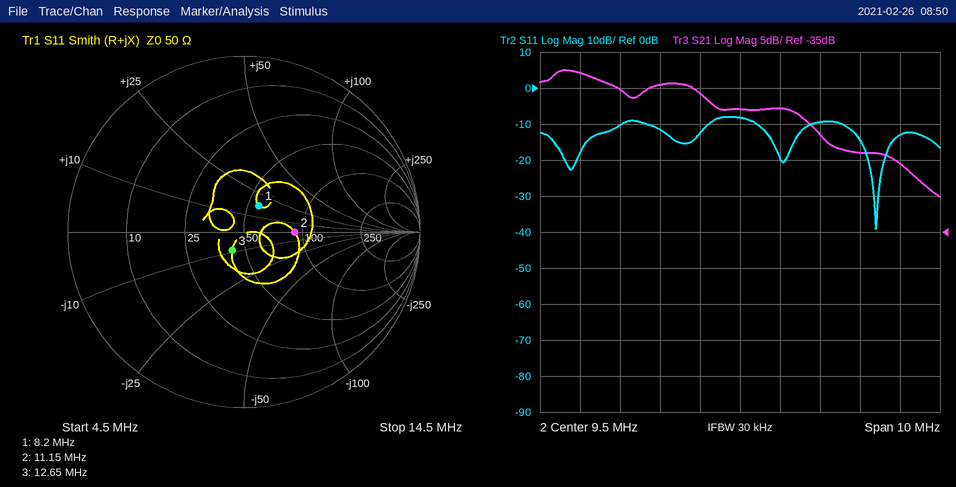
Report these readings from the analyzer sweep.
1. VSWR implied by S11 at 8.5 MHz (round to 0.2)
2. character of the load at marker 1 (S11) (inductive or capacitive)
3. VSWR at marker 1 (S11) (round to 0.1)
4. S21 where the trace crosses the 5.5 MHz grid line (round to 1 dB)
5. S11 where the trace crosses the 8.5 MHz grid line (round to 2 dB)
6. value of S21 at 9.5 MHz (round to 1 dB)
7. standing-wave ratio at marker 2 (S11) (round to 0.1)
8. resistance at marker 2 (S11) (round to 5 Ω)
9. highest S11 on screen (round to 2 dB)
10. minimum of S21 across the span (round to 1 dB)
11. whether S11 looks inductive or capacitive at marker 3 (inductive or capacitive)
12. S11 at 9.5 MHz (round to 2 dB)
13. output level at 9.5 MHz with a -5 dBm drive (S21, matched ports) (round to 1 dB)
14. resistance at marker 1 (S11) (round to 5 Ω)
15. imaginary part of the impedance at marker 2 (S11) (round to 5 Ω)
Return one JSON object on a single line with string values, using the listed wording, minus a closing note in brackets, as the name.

{"VSWR implied by S11 at 8.5 MHz": "1.6", "character of the load at marker 1 (S11)": "inductive", "VSWR at marker 1 (S11)": "1.4", "S21 where the trace crosses the 5.5 MHz grid line": "-13 dB", "S11 where the trace crosses the 8.5 MHz grid line": "-12 dB", "value of S21 at 9.5 MHz": "-18 dB", "standing-wave ratio at marker 2 (S11)": "1.8", "resistance at marker 2 (S11)": "90 Ω", "highest S11 on screen": "-8 dB", "minimum of S21 across the span": "-30 dB", "whether S11 looks inductive or capacitive at marker 3": "capacitive", "S11 at 9.5 MHz": "-8 dB", "output level at 9.5 MHz with a -5 dBm drive (S21, matched ports)": "-23 dBm", "resistance at marker 1 (S11)": "55 Ω", "imaginary part of the impedance at marker 2 (S11)": "0 Ω"}
